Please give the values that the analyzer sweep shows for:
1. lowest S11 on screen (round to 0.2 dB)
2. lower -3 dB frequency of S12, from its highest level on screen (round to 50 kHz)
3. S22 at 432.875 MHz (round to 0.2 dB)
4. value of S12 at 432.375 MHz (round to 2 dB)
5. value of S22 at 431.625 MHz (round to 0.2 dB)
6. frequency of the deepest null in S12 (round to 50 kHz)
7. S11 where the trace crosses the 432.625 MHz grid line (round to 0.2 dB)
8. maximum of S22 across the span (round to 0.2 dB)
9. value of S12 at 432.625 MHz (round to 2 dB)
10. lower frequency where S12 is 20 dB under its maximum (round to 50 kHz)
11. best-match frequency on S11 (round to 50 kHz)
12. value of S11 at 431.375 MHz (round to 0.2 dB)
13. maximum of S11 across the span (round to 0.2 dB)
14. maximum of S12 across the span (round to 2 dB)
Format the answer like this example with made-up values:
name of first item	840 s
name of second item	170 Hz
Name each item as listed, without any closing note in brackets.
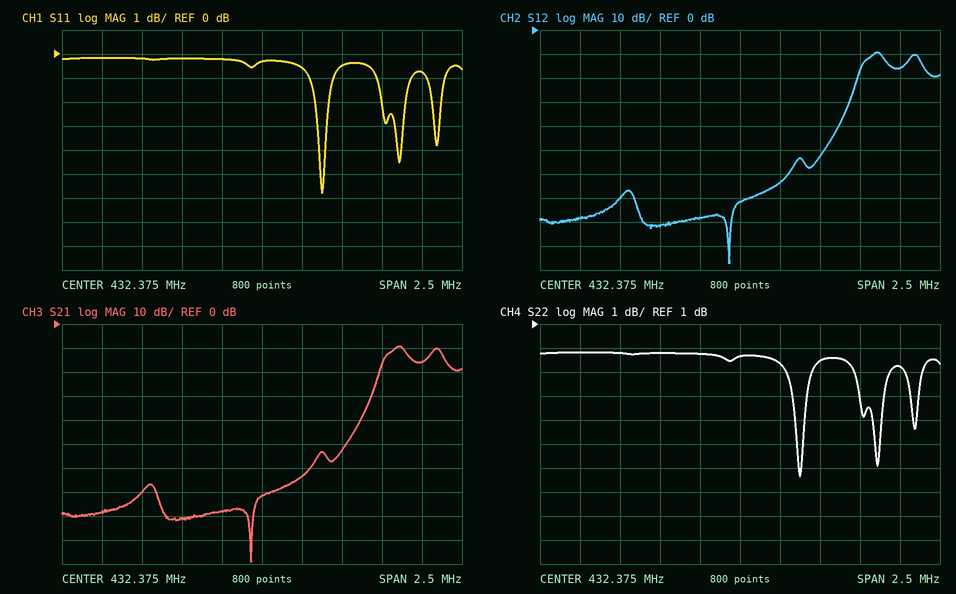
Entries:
lowest S11 on screen	-5.8 dB
lower -3 dB frequency of S12, from its highest level on screen	433.15 MHz
S22 at 432.875 MHz	-0.6 dB
value of S12 at 432.375 MHz	-72 dB
value of S22 at 431.625 MHz	-0.2 dB
frequency of the deepest null in S12	432.30 MHz
S11 where the trace crosses the 432.625 MHz grid line	-0.6 dB
maximum of S22 across the span	-0.2 dB
value of S12 at 432.625 MHz	-64 dB
lower frequency where S12 is 20 dB under its maximum	433.05 MHz
best-match frequency on S11	432.75 MHz
value of S11 at 431.375 MHz	-0.2 dB
maximum of S11 across the span	-0.2 dB
maximum of S12 across the span	-10 dB
